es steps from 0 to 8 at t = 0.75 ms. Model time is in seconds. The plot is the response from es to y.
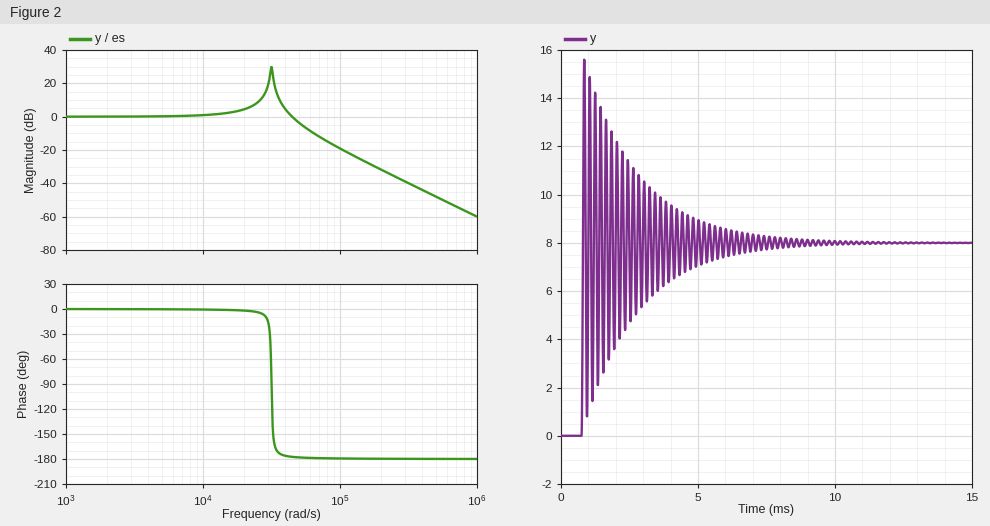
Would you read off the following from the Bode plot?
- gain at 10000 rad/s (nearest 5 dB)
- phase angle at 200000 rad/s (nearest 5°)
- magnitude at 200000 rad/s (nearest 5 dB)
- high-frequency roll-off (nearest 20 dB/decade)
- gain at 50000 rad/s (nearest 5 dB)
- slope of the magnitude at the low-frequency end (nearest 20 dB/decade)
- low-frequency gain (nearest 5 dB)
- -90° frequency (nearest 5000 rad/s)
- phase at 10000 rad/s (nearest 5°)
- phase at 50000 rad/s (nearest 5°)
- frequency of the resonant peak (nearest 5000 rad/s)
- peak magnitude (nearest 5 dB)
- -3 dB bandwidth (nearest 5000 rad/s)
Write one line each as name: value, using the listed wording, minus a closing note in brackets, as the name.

gain at 10000 rad/s: 0 dB
phase angle at 200000 rad/s: -180°
magnitude at 200000 rad/s: -30 dB
high-frequency roll-off: -40 dB/decade
gain at 50000 rad/s: -5 dB
slope of the magnitude at the low-frequency end: 0 dB/decade
low-frequency gain: 0 dB
-90° frequency: 30000 rad/s
phase at 10000 rad/s: 0°
phase at 50000 rad/s: -180°
frequency of the resonant peak: 30000 rad/s
peak magnitude: 30 dB
-3 dB bandwidth: 50000 rad/s
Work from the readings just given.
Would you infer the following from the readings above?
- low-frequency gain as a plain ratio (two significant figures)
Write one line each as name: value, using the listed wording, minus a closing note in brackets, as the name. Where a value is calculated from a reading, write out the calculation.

low-frequency gain as a plain ratio: 10^(0 / 20) = 1.0
